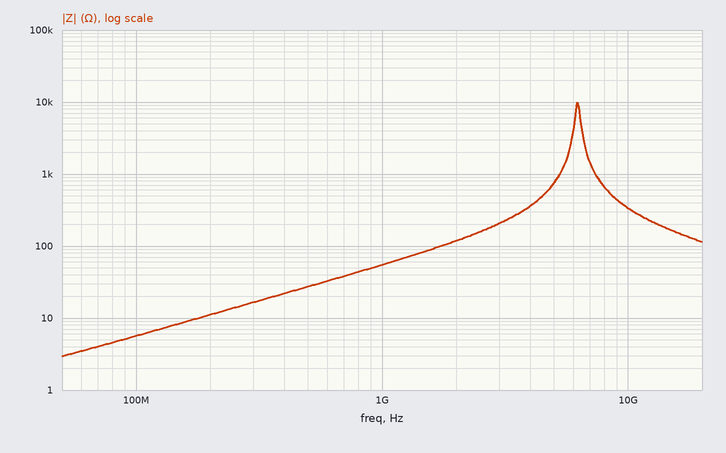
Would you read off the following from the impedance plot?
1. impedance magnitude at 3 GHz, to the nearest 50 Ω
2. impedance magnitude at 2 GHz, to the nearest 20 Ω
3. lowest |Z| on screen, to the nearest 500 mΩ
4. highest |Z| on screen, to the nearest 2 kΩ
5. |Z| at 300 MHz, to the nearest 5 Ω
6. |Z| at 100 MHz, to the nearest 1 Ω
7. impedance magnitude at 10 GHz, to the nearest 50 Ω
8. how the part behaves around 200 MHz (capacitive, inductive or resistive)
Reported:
200 Ω
120 Ω
3.0 Ω
10 kΩ
15 Ω
6 Ω
350 Ω
inductive
